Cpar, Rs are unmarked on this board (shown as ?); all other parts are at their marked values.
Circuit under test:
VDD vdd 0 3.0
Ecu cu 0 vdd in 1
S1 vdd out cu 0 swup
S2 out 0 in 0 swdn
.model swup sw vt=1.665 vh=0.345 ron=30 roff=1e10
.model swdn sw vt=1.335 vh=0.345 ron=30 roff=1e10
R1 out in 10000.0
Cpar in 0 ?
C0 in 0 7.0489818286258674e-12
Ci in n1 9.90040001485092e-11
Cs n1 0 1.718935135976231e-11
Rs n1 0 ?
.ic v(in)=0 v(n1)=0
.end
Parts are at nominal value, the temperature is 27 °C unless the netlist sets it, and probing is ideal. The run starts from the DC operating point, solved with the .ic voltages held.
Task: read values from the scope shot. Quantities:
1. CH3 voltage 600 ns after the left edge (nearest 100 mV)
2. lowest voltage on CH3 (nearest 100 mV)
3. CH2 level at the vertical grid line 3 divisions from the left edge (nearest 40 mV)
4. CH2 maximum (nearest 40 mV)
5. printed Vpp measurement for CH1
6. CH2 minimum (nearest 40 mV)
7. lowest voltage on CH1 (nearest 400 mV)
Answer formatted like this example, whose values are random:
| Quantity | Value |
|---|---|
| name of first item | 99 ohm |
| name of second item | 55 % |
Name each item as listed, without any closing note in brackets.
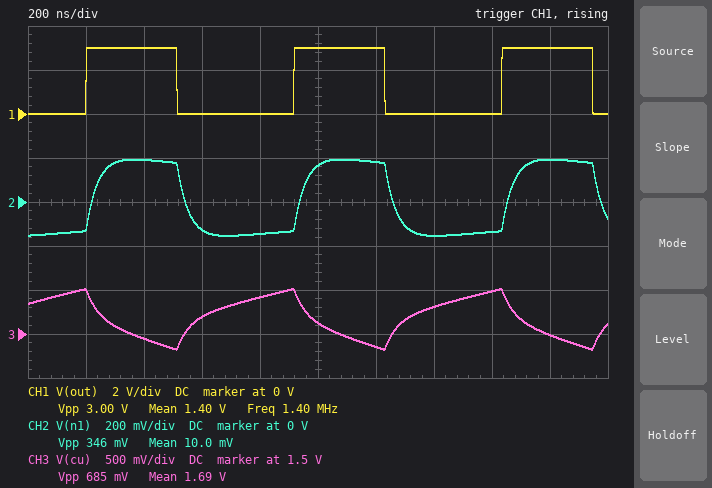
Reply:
| Quantity | Value |
|---|---|
| CH3 voltage 600 ns after the left edge | 1.7 V |
| lowest voltage on CH3 | 1.3 V |
| CH2 level at the vertical grid line 3 divisions from the left edge | -120 mV |
| CH2 maximum | 200 mV |
| printed Vpp measurement for CH1 | 3.00 V |
| CH2 minimum | -160 mV |
| lowest voltage on CH1 | 0 V |
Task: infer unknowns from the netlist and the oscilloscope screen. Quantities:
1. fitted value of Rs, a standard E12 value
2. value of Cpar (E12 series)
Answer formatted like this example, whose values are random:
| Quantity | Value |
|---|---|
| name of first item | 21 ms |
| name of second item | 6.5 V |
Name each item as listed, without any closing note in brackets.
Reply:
| Quantity | Value |
|---|---|
| fitted value of Rs, a standard E12 value | 1.5 kΩ |
| value of Cpar | 8.2 pF |
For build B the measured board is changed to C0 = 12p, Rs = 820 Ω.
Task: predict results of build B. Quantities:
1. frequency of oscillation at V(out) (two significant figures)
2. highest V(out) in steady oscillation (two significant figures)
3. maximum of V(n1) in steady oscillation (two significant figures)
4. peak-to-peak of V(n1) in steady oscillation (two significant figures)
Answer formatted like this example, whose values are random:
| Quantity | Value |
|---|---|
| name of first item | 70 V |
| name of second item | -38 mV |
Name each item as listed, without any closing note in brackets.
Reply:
| Quantity | Value |
|---|---|
| frequency of oscillation at V(out) | 1.0 MHz |
| highest V(out) in steady oscillation | 3.0 V |
| maximum of V(n1) in steady oscillation | 110 mV |
| peak-to-peak of V(n1) in steady oscillation | 210 mV |
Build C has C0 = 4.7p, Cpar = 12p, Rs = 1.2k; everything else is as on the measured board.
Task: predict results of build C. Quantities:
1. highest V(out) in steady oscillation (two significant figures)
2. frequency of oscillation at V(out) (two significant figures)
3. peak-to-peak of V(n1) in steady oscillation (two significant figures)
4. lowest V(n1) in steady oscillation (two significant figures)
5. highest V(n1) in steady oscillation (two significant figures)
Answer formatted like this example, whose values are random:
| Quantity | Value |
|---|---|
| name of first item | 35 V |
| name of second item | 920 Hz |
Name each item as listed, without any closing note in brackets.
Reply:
| Quantity | Value |
|---|---|
| highest V(out) in steady oscillation | 3.0 V |
| frequency of oscillation at V(out) | 1.2 MHz |
| peak-to-peak of V(n1) in steady oscillation | 290 mV |
| lowest V(n1) in steady oscillation | -130 mV |
| highest V(n1) in steady oscillation | 160 mV |
